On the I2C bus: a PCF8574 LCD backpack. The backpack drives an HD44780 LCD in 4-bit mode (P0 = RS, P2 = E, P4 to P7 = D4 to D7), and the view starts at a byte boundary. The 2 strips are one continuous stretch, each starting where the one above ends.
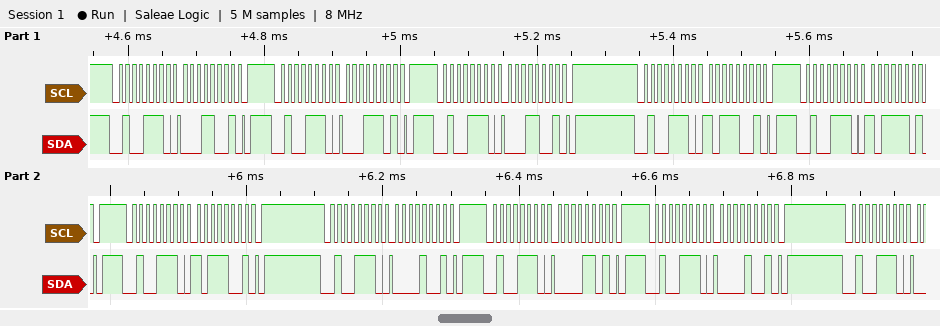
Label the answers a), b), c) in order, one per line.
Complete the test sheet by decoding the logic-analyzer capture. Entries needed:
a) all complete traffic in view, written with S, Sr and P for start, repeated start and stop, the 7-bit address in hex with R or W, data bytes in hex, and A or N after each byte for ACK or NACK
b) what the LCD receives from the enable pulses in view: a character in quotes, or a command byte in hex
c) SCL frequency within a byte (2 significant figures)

a) S 27W A 19 A P S 27W A 1D A P S 27W A 19 A P S 27W A B9 A P S 27W A BD A P S 27W A B9 A P S 27W A 09 A P S 27W A 0D A P S 27W A 09 A P S 27W A
b) data 0x1B
c) 100 kHz
